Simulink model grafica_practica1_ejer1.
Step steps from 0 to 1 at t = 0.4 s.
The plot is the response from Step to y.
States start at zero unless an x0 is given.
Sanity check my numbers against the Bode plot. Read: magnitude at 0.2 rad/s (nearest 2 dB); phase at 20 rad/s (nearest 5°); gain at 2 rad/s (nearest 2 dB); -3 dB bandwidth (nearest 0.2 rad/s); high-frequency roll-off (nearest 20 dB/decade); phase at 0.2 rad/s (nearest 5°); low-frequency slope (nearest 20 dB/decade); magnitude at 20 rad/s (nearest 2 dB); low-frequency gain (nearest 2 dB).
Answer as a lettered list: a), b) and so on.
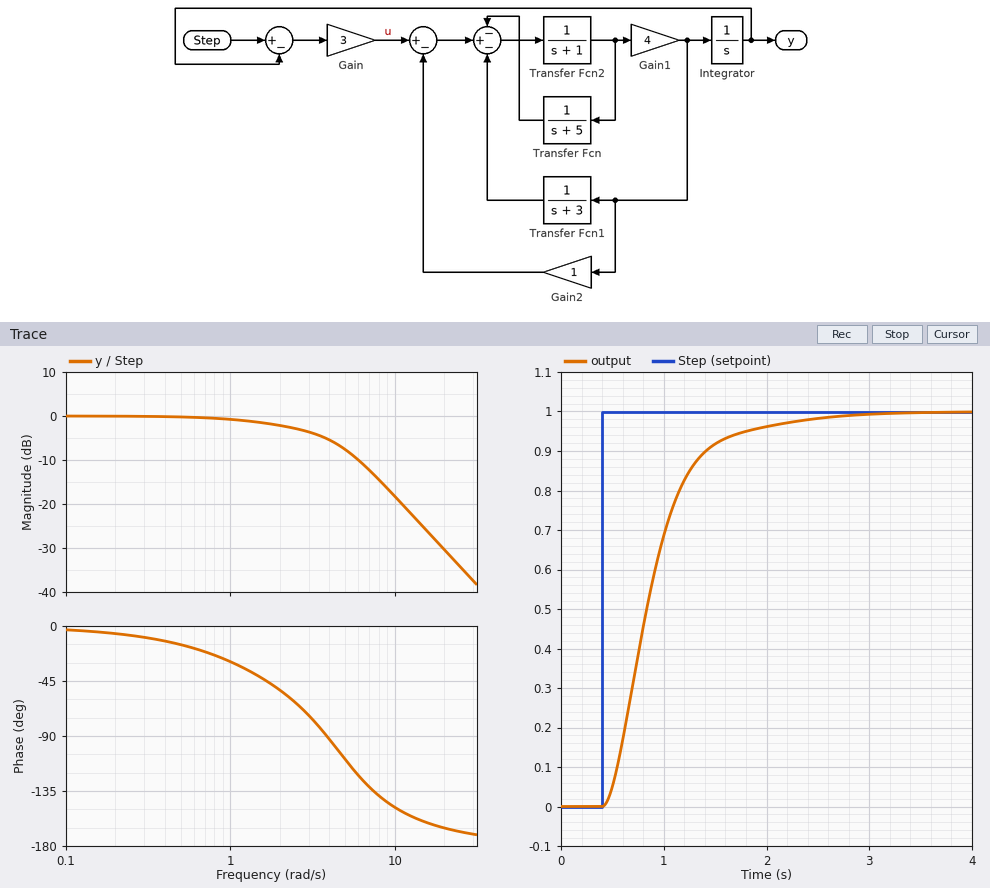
a) 0 dB
b) -165°
c) -2 dB
d) 2.6 rad/s
e) -40 dB/decade
f) -5°
g) 0 dB/decade
h) -30 dB
i) 0 dB
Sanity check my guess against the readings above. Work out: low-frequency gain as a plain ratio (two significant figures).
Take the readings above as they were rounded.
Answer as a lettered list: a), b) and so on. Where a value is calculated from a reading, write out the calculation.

a) 10^(0 / 20) = 1.0
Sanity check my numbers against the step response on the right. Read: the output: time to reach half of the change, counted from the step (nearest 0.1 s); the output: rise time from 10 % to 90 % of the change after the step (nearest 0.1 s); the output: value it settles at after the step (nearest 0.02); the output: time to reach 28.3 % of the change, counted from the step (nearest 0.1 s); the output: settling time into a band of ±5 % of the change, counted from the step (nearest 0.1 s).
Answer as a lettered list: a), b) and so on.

a) 0.4 s
b) 0.9 s
c) 1.00
d) 0.3 s
e) 1.4 s
